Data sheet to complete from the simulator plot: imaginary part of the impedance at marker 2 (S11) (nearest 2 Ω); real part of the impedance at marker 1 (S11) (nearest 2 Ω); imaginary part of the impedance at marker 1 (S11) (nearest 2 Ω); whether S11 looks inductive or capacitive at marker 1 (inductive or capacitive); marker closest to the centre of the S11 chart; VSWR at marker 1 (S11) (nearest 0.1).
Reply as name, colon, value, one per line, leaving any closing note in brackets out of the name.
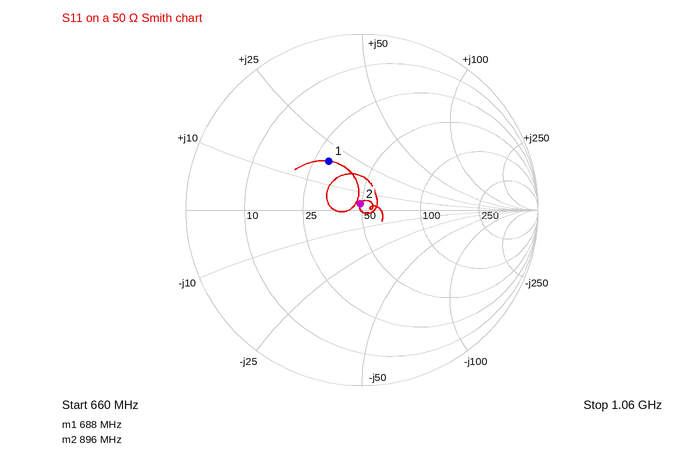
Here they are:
imaginary part of the impedance at marker 2 (S11): +4 Ω
real part of the impedance at marker 1 (S11): 30 Ω
imaginary part of the impedance at marker 1 (S11): +18 Ω
whether S11 looks inductive or capacitive at marker 1: inductive
marker closest to the centre of the S11 chart: marker 2
VSWR at marker 1 (S11): 2.0
